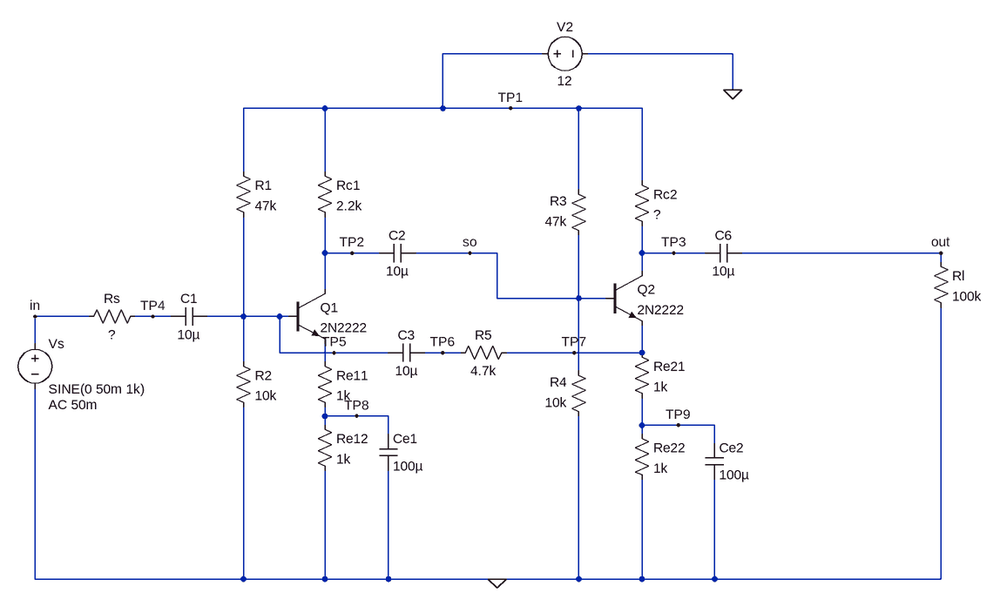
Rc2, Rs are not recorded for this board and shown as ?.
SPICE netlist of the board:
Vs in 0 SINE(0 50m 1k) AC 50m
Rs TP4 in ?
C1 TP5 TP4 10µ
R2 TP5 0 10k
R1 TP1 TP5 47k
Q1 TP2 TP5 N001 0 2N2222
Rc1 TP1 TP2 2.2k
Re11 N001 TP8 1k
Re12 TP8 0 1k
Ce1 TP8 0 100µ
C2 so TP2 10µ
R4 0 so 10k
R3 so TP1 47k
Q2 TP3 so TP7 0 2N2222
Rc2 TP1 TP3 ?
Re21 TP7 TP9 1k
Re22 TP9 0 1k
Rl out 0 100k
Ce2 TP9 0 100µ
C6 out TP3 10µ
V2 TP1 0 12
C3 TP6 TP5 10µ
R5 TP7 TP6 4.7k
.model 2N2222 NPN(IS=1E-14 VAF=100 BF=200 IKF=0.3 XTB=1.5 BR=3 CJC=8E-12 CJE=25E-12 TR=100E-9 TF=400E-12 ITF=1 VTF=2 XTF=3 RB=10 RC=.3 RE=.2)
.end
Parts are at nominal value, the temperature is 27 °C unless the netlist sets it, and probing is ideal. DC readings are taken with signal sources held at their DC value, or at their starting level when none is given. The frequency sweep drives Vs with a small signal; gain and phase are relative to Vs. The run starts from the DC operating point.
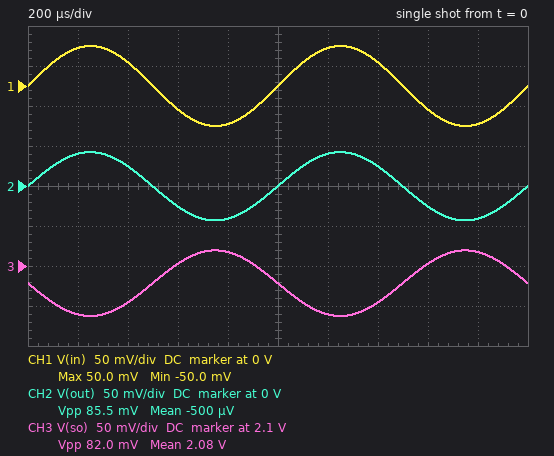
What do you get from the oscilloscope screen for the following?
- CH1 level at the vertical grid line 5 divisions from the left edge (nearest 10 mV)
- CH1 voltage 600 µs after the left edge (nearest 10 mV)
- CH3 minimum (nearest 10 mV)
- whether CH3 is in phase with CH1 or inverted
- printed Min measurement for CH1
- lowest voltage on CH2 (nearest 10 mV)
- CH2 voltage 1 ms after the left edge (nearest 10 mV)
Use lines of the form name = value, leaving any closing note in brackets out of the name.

CH1 level at the vertical grid line 5 divisions from the left edge = 0 V
CH1 voltage 600 µs after the left edge = -30 mV
CH3 minimum = 2.04 V
whether CH3 is in phase with CH1 or inverted = inverted
printed Min measurement for CH1 = -50.0 mV
lowest voltage on CH2 = -40 mV
CH2 voltage 1 ms after the left edge = 0 V
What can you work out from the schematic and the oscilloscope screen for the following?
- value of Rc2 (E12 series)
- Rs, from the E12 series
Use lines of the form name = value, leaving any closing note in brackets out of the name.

value of Rc2 = 820 Ω
Rs, from the E12 series = 1.5 kΩ
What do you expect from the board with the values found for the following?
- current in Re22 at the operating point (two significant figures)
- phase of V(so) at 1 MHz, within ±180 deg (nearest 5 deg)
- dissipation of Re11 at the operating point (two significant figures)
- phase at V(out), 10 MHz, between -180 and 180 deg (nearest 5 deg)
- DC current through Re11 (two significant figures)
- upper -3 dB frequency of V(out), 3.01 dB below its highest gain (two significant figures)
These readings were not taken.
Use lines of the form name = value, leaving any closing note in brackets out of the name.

current in Re22 at the operating point = 720 µA
phase of V(so) at 1 MHz, within ±180 deg = 170 deg
dissipation of Re11 at the operating point = 510 µW
phase at V(out), 10 MHz, between -180 and 180 deg = -95 deg
DC current through Re11 = 720 µA
upper -3 dB frequency of V(out), 3.01 dB below its highest gain = 7.3 MHz
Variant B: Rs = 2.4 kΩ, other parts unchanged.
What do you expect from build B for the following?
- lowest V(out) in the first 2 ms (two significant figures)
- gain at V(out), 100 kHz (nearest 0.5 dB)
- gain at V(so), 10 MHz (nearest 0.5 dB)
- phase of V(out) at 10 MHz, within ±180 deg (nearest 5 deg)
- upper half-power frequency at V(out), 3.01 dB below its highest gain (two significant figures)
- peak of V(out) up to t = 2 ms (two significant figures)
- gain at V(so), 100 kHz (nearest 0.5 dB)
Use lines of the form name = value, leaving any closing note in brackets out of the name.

lowest V(out) in the first 2 ms = -33 mV
gain at V(out), 100 kHz = -3.5 dB
gain at V(so), 10 MHz = -8.0 dB
phase of V(out) at 10 MHz, within ±180 deg = -100 deg
upper half-power frequency at V(out), 3.01 dB below its highest gain = 7.4 MHz
peak of V(out) up to t = 2 ms = 33 mV
gain at V(so), 100 kHz = -4.0 dB
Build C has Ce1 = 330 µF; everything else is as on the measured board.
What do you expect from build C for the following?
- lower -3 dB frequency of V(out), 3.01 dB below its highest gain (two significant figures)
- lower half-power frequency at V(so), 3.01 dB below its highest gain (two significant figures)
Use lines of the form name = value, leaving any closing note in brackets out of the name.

lower -3 dB frequency of V(out), 3.01 dB below its highest gain = 6.8 Hz
lower half-power frequency at V(so), 3.01 dB below its highest gain = 5.5 Hz
